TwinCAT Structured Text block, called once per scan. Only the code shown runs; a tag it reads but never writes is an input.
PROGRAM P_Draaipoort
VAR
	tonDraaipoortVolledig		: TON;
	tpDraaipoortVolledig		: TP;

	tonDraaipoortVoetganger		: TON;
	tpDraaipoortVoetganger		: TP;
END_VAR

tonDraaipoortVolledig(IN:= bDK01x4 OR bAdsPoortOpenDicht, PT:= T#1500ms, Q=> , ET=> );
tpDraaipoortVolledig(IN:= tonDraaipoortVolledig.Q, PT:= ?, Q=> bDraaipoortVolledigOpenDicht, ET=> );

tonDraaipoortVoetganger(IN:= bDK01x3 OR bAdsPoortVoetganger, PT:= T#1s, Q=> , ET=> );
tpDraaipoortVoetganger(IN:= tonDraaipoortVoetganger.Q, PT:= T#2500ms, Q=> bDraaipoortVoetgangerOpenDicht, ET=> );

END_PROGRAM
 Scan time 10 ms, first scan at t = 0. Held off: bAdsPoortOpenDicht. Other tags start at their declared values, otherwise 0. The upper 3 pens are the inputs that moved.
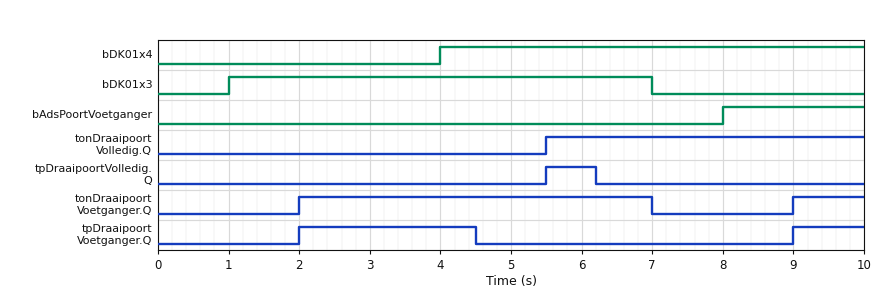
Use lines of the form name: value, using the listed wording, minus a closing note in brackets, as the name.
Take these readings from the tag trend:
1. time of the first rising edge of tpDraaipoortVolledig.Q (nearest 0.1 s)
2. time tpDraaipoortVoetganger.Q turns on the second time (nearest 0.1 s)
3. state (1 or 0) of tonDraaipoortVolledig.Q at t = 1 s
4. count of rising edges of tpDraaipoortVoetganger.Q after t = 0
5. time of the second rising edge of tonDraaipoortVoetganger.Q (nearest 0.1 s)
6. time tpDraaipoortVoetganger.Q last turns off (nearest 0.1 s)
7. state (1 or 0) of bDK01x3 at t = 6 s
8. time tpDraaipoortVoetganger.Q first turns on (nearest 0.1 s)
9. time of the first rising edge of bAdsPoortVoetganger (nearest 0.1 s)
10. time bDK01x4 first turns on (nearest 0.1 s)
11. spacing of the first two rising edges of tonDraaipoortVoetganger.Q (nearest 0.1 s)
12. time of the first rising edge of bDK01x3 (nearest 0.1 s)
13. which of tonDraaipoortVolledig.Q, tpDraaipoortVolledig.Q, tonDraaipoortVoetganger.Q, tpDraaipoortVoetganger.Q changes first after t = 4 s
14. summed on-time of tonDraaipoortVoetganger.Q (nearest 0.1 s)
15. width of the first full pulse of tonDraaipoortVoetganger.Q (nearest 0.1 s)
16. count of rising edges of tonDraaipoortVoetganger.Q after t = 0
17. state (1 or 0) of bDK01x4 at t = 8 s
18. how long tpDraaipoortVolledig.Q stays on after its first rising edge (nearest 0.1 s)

time of the first rising edge of tpDraaipoortVolledig.Q: 5.5 s
time tpDraaipoortVoetganger.Q turns on the second time: 9.0 s
state (1 or 0) of tonDraaipoortVolledig.Q at t = 1 s: 0
count of rising edges of tpDraaipoortVoetganger.Q after t = 0: 2
time of the second rising edge of tonDraaipoortVoetganger.Q: 9.0 s
time tpDraaipoortVoetganger.Q last turns off: 4.5 s
state (1 or 0) of bDK01x3 at t = 6 s: 1
time tpDraaipoortVoetganger.Q first turns on: 2.0 s
time of the first rising edge of bAdsPoortVoetganger: 8.0 s
time bDK01x4 first turns on: 4.0 s
spacing of the first two rising edges of tonDraaipoortVoetganger.Q: 7.0 s
time of the first rising edge of bDK01x3: 1.0 s
which of tonDraaipoortVolledig.Q, tpDraaipoortVolledig.Q, tonDraaipoortVoetganger.Q, tpDraaipoortVoetganger.Q changes first after t = 4 s: tpDraaipoortVoetganger.Q
summed on-time of tonDraaipoortVoetganger.Q: 6.0 s
width of the first full pulse of tonDraaipoortVoetganger.Q: 5.0 s
count of rising edges of tonDraaipoortVoetganger.Q after t = 0: 2
state (1 or 0) of bDK01x4 at t = 8 s: 1
how long tpDraaipoortVolledig.Q stays on after its first rising edge: 0.7 s
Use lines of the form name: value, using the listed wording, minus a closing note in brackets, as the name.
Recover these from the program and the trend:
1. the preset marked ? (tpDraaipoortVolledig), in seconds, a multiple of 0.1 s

the preset marked ? (tpDraaipoortVolledig), in seconds, a multiple of 0.1 s: 0.7 s
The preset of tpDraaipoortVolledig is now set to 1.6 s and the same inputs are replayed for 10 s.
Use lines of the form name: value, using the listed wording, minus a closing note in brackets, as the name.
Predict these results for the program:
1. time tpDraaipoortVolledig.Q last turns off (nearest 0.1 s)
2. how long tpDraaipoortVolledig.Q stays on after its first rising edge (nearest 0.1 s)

time tpDraaipoortVolledig.Q last turns off: 7.1 s
how long tpDraaipoortVolledig.Q stays on after its first rising edge: 1.6 s
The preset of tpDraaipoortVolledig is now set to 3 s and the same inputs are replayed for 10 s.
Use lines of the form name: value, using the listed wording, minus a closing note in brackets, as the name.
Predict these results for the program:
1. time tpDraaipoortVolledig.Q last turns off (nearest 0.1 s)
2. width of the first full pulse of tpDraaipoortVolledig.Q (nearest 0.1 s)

time tpDraaipoortVolledig.Q last turns off: 8.5 s
width of the first full pulse of tpDraaipoortVolledig.Q: 3.0 s
